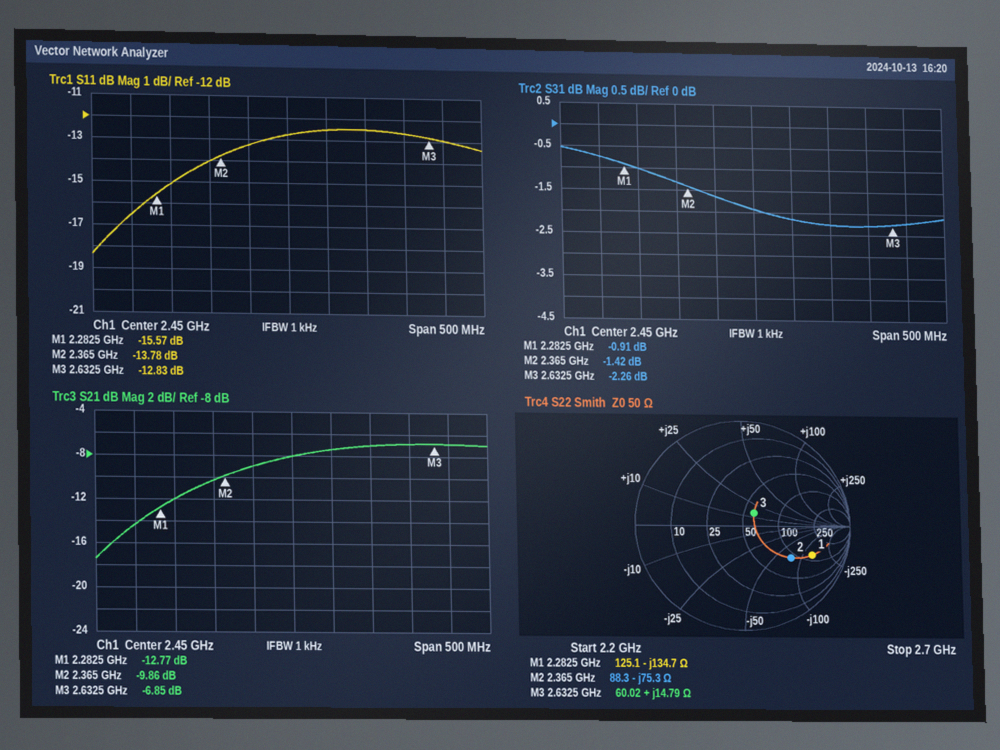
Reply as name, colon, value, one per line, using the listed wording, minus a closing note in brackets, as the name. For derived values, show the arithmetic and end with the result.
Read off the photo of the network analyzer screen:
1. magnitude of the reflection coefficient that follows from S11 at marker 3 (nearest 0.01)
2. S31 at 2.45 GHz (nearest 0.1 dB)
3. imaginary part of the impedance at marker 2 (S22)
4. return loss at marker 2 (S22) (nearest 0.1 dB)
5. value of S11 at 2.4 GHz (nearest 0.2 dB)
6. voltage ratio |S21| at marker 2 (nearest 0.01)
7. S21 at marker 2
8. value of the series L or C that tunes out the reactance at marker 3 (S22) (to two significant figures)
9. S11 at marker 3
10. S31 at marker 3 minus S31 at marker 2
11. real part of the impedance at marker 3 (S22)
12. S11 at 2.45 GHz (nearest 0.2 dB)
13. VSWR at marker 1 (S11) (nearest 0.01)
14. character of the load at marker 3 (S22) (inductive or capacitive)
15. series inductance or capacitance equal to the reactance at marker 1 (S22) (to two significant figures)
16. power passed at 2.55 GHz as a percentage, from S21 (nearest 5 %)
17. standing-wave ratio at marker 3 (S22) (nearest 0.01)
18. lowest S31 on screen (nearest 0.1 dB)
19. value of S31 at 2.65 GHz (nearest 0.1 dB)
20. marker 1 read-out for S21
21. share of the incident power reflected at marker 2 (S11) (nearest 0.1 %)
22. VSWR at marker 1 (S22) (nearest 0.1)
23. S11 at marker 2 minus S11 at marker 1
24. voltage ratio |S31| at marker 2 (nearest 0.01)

magnitude of the reflection coefficient that follows from S11 at marker 3: 10^(-12.83/20) ≈ 0.23
S31 at 2.45 GHz: -1.9 dB
imaginary part of the impedance at marker 2: -75.3 Ω
return loss at marker 2 (S22): 5.4 dB
value of S11 at 2.4 GHz: -13.2 dB
voltage ratio |S21| at marker 2: 10^(-9.86/20) ≈ 0.32
S21 at marker 2: -9.86 dB
value of the series L or C that tunes out the reactance at marker 3 (S22): C = 1/(2π × 2.6325 GHz × 14.79 Ω) ≈ 4.1 pF
S11 at marker 3: -12.83 dB
S31 at marker 3 minus S31 at marker 2: -2.26 − (-1.42) = -0.84 dB
real part of the impedance at marker 3: 60.02 Ω
S11 at 2.45 GHz: -12.8 dB
VSWR at marker 1 (S11): (1 + 0.1665)/(1 − 0.1665) ≈ 1.40
character of the load at marker 3 (S22): inductive
series inductance or capacitance equal to the reactance at marker 1 (S22): C = 1/(2π × 2.2825 GHz × 134.7 Ω) ≈ 518 fF, so 520 fF to two significant figures
power passed at 2.55 GHz as a percentage, from S21: 10^(-7/10) ≈ 20 %
standing-wave ratio at marker 3 (S22): 1.38
lowest S31 on screen: -2.3 dB
value of S31 at 2.65 GHz: -2.2 dB
marker 1 read-out for S21: -12.77 dB
share of the incident power reflected at marker 2 (S11): 10^(-13.78/10) ≈ 4.2 %
VSWR at marker 1 (S22): 5.6
S11 at marker 2 minus S11 at marker 1: -13.78 − (-15.57) = 1.79 dB
voltage ratio |S31| at marker 2: 10^(-1.42/20) ≈ 0.85
